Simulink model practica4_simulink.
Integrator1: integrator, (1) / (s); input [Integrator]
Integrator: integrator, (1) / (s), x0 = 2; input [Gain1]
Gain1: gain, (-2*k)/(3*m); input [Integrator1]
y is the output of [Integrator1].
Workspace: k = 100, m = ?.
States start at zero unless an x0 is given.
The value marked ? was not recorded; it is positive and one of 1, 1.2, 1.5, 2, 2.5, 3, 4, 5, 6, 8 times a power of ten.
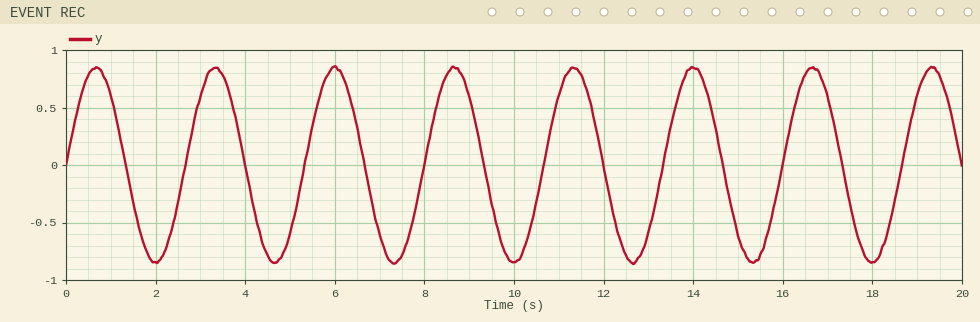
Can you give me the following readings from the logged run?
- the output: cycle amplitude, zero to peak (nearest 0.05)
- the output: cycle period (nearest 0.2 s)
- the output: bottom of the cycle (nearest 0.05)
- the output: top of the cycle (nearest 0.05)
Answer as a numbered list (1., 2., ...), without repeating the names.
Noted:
1. 0.85
2. 2.6 s
3. -0.85
4. 0.85
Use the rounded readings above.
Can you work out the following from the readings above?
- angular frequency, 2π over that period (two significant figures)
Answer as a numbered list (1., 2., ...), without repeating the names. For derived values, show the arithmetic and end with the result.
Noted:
1. 2π / 2.6 = 2.4 rad/s
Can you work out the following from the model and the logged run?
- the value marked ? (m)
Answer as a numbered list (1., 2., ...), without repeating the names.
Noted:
1. 12
